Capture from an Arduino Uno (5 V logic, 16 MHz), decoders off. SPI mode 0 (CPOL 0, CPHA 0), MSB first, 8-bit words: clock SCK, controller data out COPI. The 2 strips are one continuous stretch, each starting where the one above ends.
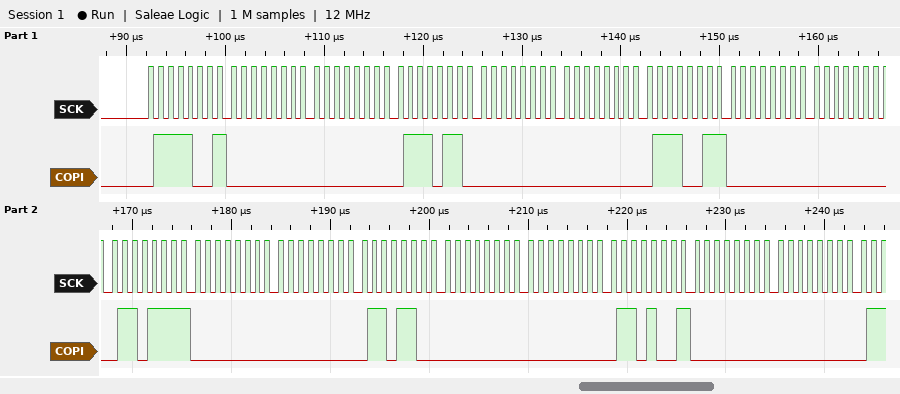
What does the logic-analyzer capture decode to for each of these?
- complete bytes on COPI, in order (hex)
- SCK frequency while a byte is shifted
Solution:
0x79 0x00 0x00 0x76 0x00 0x00 0x73 0x00 0x00 0x6F 0x00 0x00 0x6C 0x00 0x00 0x69 0x00 0x00
1 MHz
